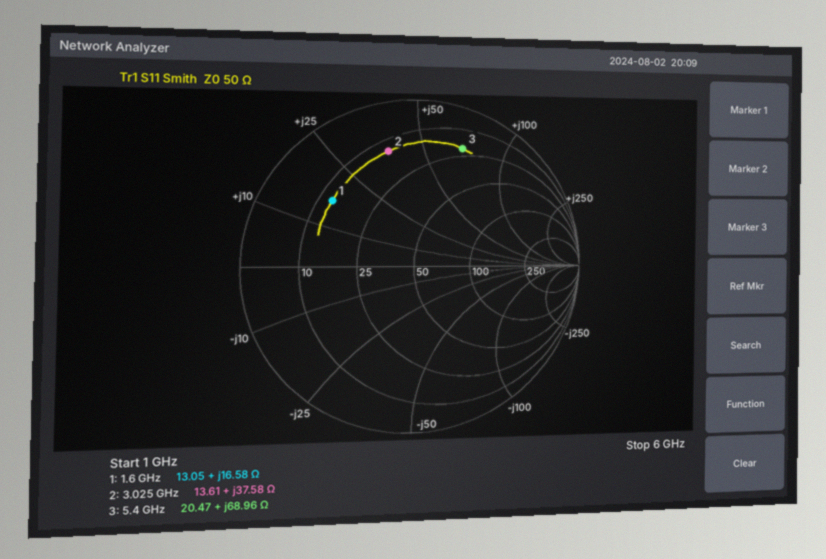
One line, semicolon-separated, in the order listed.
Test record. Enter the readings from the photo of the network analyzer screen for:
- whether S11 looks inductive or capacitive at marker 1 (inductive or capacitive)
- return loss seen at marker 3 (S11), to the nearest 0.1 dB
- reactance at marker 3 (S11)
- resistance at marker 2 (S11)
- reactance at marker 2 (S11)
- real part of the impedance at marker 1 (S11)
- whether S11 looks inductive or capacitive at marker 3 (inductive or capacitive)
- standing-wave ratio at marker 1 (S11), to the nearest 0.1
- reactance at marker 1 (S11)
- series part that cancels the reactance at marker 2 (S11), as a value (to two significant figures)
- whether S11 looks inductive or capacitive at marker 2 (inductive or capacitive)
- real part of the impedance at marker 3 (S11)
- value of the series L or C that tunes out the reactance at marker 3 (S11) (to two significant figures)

inductive; 2.4 dB; +68.96 Ω; 13.61 Ω; +37.58 Ω; 13.05 Ω; inductive; 4.3; +16.58 Ω; 1.4 pF; inductive; 20.47 Ω; 430 fF
